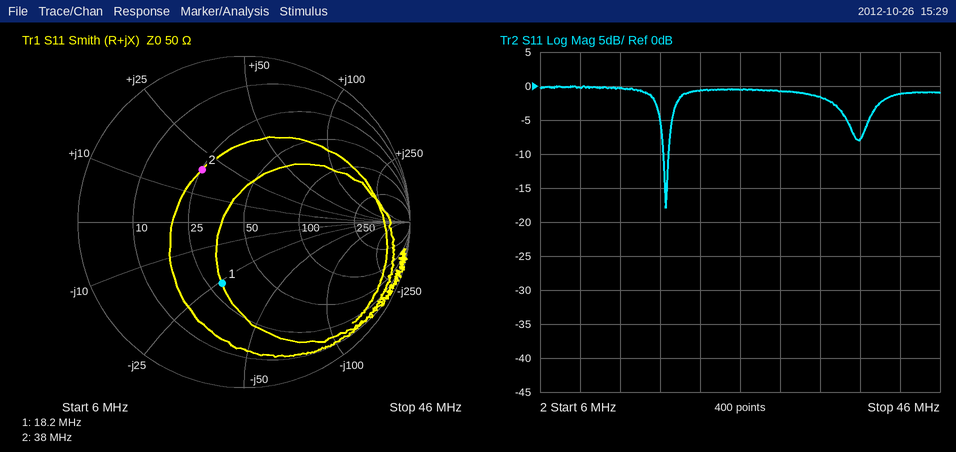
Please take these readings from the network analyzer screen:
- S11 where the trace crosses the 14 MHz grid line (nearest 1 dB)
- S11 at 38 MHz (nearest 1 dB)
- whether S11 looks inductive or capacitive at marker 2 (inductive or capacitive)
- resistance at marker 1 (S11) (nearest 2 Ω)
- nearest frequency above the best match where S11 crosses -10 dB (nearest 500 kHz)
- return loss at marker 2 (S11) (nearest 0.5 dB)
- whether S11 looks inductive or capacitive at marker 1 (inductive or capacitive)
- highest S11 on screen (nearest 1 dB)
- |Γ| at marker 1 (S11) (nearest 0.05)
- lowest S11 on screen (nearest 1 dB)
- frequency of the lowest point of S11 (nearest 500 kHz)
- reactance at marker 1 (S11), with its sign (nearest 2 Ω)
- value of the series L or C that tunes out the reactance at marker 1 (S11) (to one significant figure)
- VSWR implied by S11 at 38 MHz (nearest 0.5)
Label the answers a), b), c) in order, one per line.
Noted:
a) 0 dB
b) -8 dB
c) inductive
d) 30 Ω
e) 19.0 MHz
f) 8.0 dB
g) capacitive
h) 0 dB
i) 0.40
j) -18 dB
k) 18.5 MHz
l) -26 Ω
m) 200 nH
n) 2.5
